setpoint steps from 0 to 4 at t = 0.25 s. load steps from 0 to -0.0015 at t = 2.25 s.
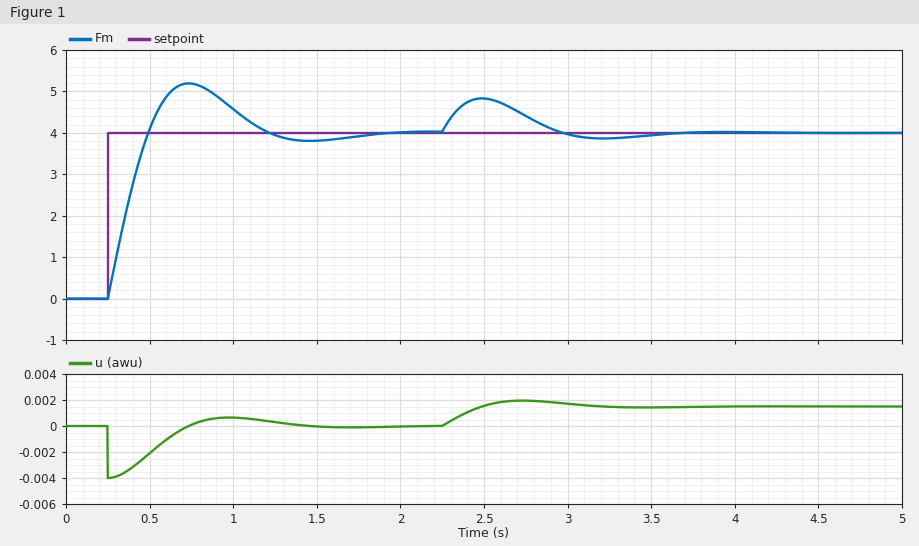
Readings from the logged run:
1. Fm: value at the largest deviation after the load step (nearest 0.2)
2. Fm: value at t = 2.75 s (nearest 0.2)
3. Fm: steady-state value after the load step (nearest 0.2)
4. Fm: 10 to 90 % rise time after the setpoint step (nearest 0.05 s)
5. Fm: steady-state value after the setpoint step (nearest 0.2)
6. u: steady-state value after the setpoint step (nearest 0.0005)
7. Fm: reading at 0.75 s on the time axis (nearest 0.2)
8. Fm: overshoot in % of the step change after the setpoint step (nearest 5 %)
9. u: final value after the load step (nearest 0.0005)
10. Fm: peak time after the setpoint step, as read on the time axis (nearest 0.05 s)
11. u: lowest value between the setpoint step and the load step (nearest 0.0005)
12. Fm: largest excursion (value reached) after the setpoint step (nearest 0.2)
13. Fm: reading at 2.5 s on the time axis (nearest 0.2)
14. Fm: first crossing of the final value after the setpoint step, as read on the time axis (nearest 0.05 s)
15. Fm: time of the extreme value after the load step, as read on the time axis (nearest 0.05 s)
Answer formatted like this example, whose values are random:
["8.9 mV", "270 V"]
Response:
["4.8", "4.4", "4.0", "0.20 s", "4.0", "0.0000", "5.2", "30 %", "0.0015", "0.75 s", "-0.0040", "5.2", "4.8", "0.50 s", "2.50 s"]
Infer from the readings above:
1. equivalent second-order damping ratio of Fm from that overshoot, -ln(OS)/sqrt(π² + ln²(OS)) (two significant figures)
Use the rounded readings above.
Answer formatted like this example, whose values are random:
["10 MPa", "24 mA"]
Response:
["0.36"]
